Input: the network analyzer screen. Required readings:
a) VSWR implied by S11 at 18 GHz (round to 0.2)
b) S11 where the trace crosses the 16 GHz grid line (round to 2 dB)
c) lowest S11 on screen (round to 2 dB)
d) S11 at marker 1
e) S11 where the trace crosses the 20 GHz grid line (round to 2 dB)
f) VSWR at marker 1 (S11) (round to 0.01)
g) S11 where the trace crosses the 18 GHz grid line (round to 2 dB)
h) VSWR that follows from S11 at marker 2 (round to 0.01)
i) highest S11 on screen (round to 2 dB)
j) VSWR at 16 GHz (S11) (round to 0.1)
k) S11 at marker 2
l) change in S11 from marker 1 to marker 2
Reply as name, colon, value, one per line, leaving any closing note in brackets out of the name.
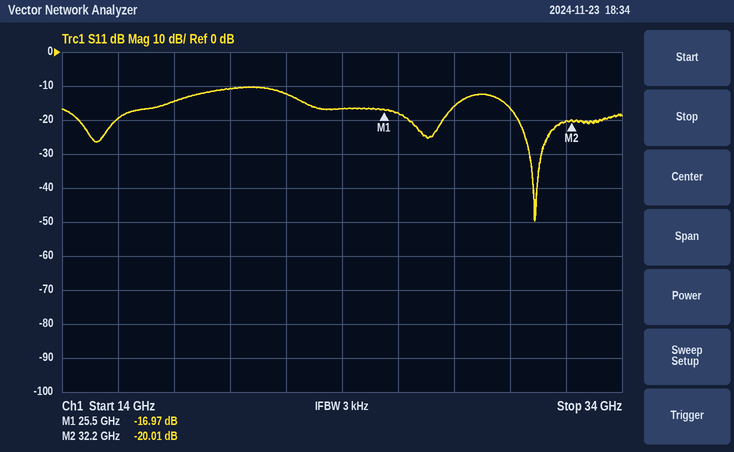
VSWR implied by S11 at 18 GHz: 1.4
S11 where the trace crosses the 16 GHz grid line: -20 dB
lowest S11 on screen: -50 dB
S11 at marker 1: -16.97 dB
S11 where the trace crosses the 20 GHz grid line: -10 dB
VSWR at marker 1 (S11): 1.33
S11 where the trace crosses the 18 GHz grid line: -14 dB
VSWR that follows from S11 at marker 2: 1.22
highest S11 on screen: -10 dB
VSWR at 16 GHz (S11): 1.2
S11 at marker 2: -20.01 dB
change in S11 from marker 1 to marker 2: -3.04 dB
